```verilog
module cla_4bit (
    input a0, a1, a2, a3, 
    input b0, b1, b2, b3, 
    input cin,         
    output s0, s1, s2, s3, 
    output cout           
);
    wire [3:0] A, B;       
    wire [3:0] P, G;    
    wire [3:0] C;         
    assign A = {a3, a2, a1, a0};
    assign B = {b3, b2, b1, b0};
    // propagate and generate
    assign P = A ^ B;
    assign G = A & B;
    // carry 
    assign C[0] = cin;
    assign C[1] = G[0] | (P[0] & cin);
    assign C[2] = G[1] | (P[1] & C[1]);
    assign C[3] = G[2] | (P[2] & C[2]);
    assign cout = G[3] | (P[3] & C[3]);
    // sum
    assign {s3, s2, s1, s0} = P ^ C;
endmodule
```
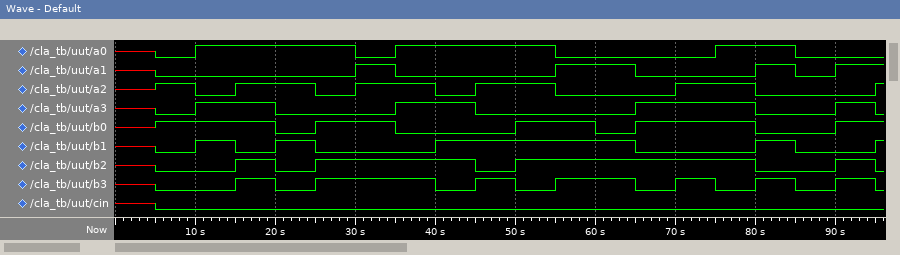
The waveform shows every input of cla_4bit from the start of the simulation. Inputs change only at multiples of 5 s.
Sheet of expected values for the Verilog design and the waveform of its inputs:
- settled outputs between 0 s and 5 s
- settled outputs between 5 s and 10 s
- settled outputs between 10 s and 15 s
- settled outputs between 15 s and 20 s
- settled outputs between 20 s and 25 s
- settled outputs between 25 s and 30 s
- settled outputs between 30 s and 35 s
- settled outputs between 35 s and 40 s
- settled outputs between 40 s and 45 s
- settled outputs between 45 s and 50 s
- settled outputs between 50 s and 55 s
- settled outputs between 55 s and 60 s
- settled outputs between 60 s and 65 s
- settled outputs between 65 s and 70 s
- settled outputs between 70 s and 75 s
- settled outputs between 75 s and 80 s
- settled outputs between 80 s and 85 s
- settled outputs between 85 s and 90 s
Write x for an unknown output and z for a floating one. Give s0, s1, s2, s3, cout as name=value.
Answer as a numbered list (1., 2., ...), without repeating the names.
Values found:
1. s0=x, s1=x, s2=x, s3=x, cout=x
2. s0=1, s1=0, s2=1, s3=0, cout=0
3. s0=0, s1=0, s2=1, s3=1, cout=0
4. s0=0, s1=1, s2=0, s3=1, cout=1
5. s0=1, s1=1, s2=1, s3=0, cout=0
6. s0=0, s1=1, s2=1, s3=1, cout=0
7. s0=1, s1=1, s2=0, s3=0, cout=1
8. s0=1, s1=0, s2=0, s3=1, cout=1
9. s0=1, s1=1, s2=1, s3=1, cout=0
10. s0=1, s1=1, s2=1, s3=1, cout=0
11. s0=0, s1=0, s2=1, s3=1, cout=0
12. s0=1, s1=0, s2=0, s3=0, cout=1
13. s0=0, s1=0, s2=0, s3=0, cout=1
14. s0=1, s1=0, s2=1, s3=1, cout=0
15. s0=1, s1=0, s2=0, s3=1, cout=1
16. s0=0, s1=1, s2=0, s3=0, cout=1
17. s0=1, s1=0, s2=1, s3=1, cout=0
18. s0=0, s1=0, s2=0, s3=0, cout=0
